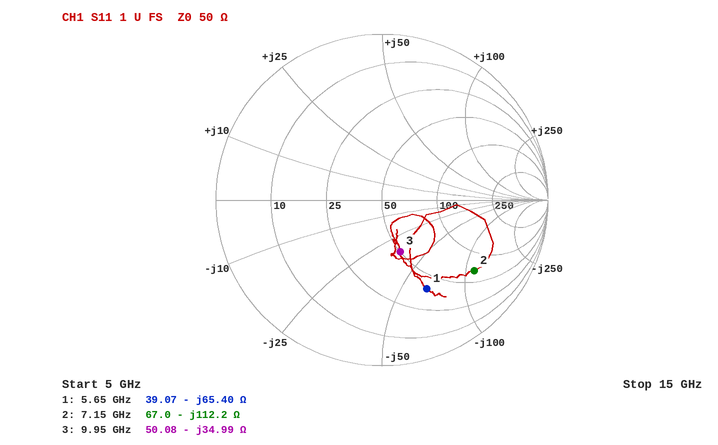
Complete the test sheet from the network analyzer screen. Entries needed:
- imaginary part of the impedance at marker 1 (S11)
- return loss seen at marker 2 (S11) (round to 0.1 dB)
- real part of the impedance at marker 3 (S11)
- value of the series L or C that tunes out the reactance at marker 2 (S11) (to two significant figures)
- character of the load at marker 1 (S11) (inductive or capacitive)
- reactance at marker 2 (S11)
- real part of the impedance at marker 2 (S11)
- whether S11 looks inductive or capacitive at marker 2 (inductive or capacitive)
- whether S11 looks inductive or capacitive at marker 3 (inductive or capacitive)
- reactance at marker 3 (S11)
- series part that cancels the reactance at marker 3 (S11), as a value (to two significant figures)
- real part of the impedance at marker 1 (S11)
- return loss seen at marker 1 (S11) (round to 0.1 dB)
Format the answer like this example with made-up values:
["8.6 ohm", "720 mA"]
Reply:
["-65.40 Ω", "3.1 dB", "50.08 Ω", "2.5 nH", "capacitive", "-112.2 Ω", "67.0 Ω", "capacitive", "capacitive", "-34.99 Ω", "560 pH", "39.07 Ω", "4.4 dB"]
